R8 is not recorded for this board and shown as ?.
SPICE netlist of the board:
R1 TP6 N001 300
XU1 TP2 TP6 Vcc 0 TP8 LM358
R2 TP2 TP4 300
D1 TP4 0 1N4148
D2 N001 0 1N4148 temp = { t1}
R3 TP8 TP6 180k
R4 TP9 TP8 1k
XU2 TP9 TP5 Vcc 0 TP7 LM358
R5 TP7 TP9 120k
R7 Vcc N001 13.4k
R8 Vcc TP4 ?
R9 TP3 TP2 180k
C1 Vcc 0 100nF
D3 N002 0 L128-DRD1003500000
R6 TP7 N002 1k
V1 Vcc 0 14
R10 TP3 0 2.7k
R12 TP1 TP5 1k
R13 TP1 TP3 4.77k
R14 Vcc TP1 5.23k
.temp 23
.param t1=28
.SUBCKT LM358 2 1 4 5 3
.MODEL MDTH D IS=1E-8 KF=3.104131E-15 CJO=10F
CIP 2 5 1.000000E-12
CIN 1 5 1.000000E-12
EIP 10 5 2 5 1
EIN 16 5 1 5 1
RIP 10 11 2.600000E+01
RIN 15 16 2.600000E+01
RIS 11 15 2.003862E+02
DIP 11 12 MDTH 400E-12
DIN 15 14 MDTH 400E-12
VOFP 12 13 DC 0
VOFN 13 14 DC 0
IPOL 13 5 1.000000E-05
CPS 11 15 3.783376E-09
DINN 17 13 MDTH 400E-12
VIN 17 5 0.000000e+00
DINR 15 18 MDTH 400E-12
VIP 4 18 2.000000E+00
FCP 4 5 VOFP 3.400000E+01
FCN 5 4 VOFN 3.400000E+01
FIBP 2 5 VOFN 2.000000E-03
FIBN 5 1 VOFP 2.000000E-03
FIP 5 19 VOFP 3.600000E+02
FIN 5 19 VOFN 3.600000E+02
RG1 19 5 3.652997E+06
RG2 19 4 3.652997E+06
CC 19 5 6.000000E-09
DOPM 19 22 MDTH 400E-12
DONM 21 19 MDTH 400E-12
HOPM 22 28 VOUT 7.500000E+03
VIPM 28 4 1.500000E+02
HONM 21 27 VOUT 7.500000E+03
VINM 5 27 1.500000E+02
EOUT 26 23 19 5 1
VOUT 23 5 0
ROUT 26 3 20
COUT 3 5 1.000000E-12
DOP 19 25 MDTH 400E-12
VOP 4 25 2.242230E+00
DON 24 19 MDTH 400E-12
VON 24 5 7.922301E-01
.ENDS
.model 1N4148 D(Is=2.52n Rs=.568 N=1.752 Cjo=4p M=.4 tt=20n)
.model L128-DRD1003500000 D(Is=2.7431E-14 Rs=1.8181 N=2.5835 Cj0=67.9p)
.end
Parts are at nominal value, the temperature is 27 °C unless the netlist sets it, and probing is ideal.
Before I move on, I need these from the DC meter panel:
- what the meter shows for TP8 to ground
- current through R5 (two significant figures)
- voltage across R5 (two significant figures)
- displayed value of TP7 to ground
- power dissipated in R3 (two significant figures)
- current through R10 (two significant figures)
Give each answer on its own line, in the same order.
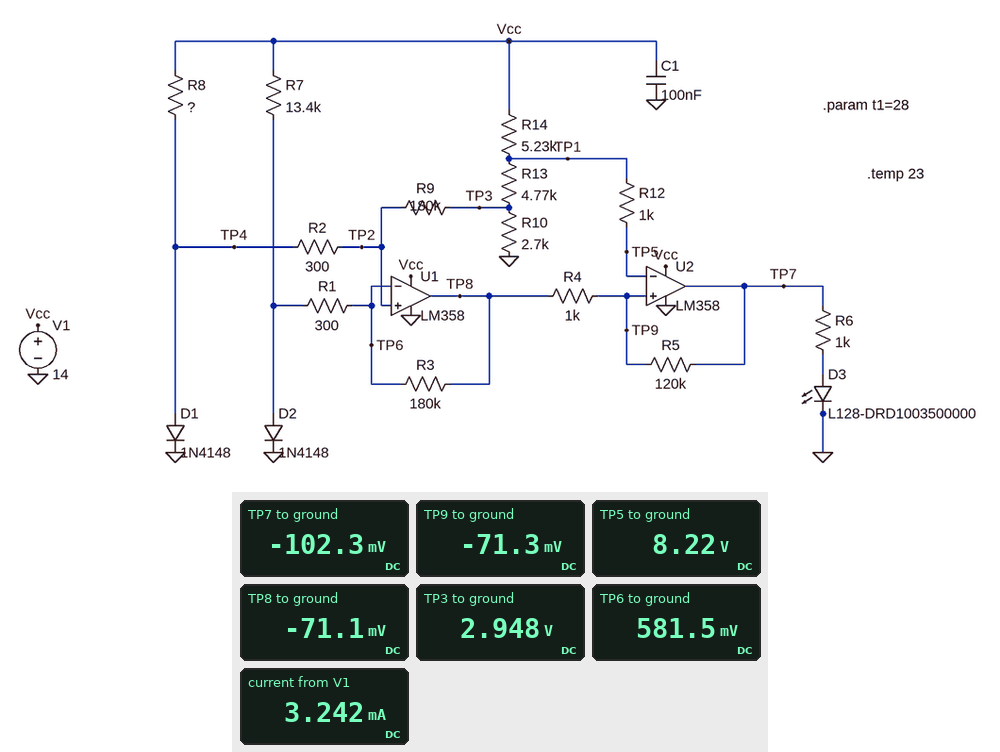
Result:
-71.1 mV
260 nA
31 mV
-102.3 mV
2.4 µW
1.1 mA
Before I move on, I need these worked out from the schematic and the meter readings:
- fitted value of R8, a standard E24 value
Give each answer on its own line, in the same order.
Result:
30 kΩ
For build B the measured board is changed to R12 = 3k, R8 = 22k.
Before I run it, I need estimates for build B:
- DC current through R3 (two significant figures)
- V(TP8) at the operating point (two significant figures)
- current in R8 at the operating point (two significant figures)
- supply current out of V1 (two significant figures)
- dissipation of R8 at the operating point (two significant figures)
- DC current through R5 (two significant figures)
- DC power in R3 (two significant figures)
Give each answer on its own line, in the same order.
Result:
3.5 µA
-42 mV
610 µA
3.4 mA
8.2 mW
500 nA
2.2 µW
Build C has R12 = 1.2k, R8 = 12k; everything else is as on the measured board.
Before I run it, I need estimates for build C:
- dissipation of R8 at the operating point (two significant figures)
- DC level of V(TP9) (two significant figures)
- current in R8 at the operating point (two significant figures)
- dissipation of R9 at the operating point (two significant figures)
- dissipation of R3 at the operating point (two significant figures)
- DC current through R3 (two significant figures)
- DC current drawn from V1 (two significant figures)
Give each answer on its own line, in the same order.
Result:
15 mW
11 V
1.1 mA
31 µW
570 µW
56 µA
310 µA
